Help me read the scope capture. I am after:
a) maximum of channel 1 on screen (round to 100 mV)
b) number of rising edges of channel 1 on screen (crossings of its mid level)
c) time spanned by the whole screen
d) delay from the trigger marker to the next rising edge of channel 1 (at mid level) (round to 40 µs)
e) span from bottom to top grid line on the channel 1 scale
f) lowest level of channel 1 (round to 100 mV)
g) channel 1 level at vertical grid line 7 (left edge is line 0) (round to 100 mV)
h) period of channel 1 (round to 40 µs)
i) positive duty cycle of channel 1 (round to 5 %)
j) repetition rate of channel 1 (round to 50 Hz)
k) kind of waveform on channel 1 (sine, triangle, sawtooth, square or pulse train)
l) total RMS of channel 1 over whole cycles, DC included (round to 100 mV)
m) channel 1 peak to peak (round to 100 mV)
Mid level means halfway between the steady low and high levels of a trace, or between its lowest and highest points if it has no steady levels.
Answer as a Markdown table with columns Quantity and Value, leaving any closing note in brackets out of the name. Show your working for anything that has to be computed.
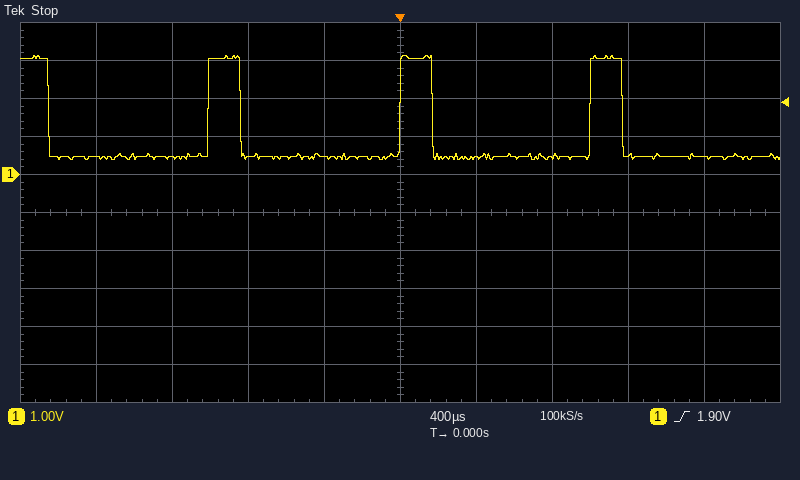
| Quantity | Value |
|---|---|
| maximum of channel 1 on screen | 3.1 V |
| number of rising edges of channel 1 on screen | 3 |
| time spanned by the whole screen | 4 ms |
| delay from the trigger marker to the next rising edge of channel 1 (at mid level) | 1.00 ms |
| span from bottom to top grid line on the channel 1 scale | 10 V |
| lowest level of channel 1 | 400 mV |
| channel 1 level at vertical grid line 7 (left edge is line 0) | 500 mV |
| period of channel 1 | 1.00 ms |
| positive duty cycle of channel 1 | 15 % |
| repetition rate of channel 1 | 1 / 1.00 ms ≈ 1.00 kHz |
| kind of waveform on channel 1 | pulse train |
| total RMS of channel 1 over whole cycles, DC included | √(0.15 × (3.1 V)² + 0.85 × (400 mV)²) ≈ 1.3 V |
| channel 1 peak to peak | 3.1 V − (400 mV) = 2.7 V |
